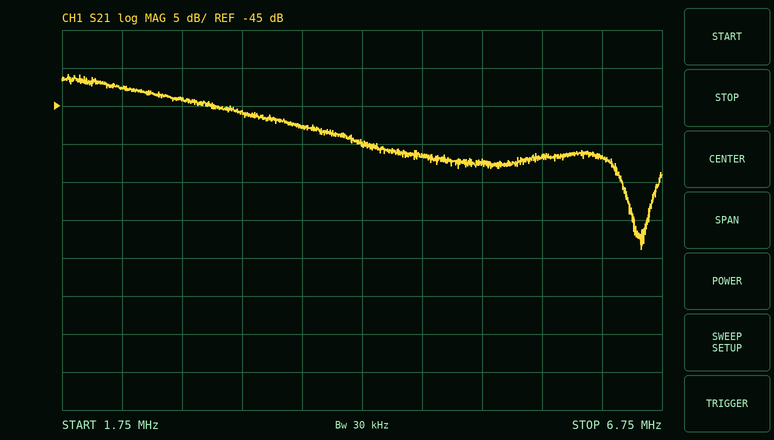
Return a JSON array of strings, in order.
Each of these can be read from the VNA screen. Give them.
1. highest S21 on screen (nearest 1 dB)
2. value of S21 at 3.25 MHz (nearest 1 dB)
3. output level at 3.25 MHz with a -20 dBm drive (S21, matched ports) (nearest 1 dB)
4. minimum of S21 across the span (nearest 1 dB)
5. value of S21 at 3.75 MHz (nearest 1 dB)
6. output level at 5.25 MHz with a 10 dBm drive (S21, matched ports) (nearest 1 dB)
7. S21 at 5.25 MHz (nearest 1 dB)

["-41 dB", "-46 dB", "-66 dBm", "-64 dB", "-48 dB", "-42 dBm", "-52 dB"]
